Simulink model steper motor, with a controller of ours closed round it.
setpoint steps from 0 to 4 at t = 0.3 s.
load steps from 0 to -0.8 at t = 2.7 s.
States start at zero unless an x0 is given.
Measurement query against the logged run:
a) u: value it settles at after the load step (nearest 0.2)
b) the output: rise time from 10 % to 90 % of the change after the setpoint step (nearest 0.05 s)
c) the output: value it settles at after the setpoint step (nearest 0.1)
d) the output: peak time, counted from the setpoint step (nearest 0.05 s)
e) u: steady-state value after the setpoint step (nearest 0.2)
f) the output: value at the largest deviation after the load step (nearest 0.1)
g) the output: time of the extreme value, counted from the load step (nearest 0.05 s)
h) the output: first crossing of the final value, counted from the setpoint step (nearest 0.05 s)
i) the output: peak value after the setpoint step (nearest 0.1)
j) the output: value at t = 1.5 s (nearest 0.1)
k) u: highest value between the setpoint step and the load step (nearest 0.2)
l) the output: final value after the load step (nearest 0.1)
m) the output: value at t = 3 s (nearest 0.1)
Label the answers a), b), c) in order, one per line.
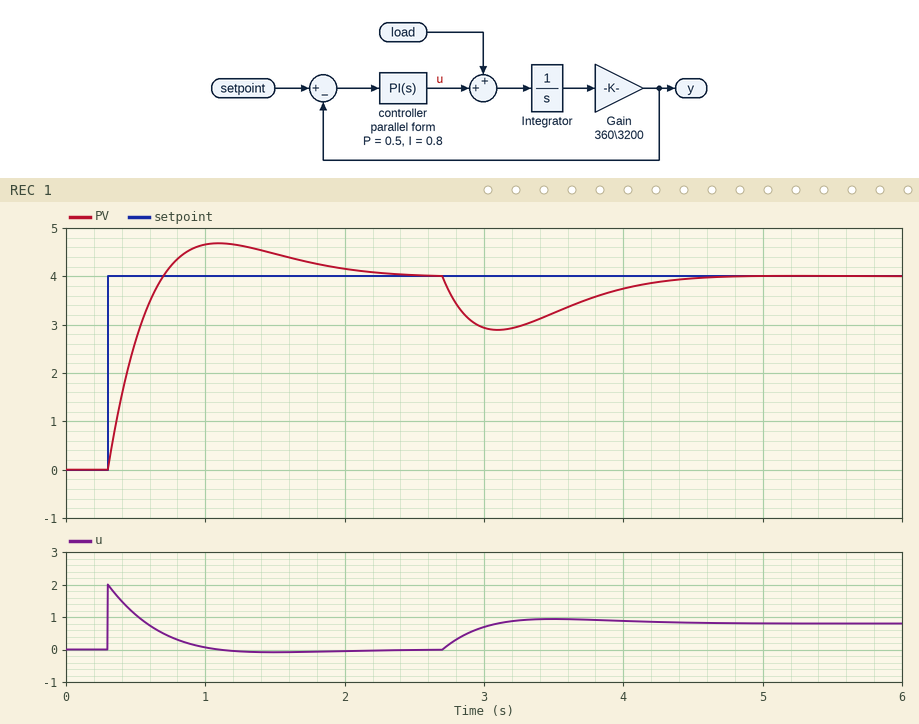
a) 0.8
b) 0.30 s
c) 4.0
d) 0.80 s
e) 0.0
f) 2.9
g) 0.40 s
h) 0.40 s
i) 4.7
j) 4.5
k) 2.0
l) 4.0
m) 2.9
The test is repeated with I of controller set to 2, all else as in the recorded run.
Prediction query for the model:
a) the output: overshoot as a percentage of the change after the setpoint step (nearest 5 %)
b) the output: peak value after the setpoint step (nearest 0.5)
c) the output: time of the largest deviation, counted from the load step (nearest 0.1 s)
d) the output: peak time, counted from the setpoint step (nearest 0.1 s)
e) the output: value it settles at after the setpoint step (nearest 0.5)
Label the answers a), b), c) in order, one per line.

a) 30 %
b) 5.0
c) 0.3 s
d) 0.6 s
e) 4.0
